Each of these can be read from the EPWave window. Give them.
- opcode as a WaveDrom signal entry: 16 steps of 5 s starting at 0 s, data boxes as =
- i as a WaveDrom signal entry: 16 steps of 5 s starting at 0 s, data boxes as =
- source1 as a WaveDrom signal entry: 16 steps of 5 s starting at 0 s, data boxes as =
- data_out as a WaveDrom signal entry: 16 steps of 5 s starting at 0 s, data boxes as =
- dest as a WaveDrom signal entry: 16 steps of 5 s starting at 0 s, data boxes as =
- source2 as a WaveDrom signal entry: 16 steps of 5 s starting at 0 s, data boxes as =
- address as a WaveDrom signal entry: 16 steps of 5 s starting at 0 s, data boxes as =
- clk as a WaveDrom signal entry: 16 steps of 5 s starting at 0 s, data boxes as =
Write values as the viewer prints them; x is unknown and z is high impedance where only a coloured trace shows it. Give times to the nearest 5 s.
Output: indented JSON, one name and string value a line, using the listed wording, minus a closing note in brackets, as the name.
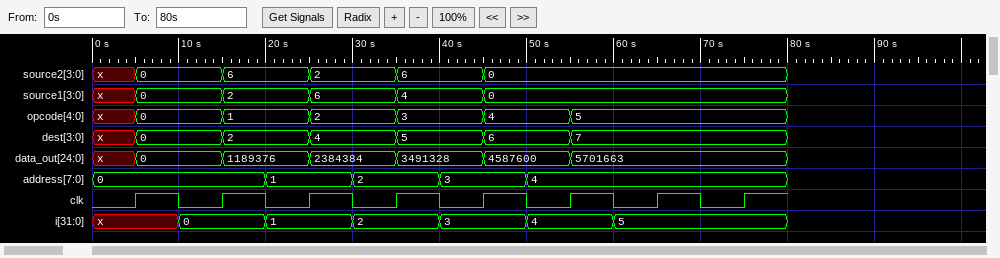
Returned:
{
  "opcode as a WaveDrom signal entry: 16 steps of 5 s starting at 0 s, data boxes as =": "{name: 'opcode', wave: 'x=.=.=.=.=.=....', data: '0 1 2 3 4 5'}",
  "i as a WaveDrom signal entry: 16 steps of 5 s starting at 0 s, data boxes as =": "{name: 'i', wave: 'x.=.=.=.=.=.=...', data: '0 1 2 3 4 5'}",
  "source1 as a WaveDrom signal entry: 16 steps of 5 s starting at 0 s, data boxes as =": "{name: 'source1', wave: 'x=.=.=.=.=......', data: '0 2 6 4 0'}",
  "data_out as a WaveDrom signal entry: 16 steps of 5 s starting at 0 s, data boxes as =": "{name: 'data_out', wave: 'x=.=.=.=.=.=....', data: '0 1189376 2384384 3491328 4587600 5701663'}",
  "dest as a WaveDrom signal entry: 16 steps of 5 s starting at 0 s, data boxes as =": "{name: 'dest', wave: 'x=.=.=.=.=.=....', data: '0 2 4 5 6 7'}",
  "source2 as a WaveDrom signal entry: 16 steps of 5 s starting at 0 s, data boxes as =": "{name: 'source2', wave: 'x=.=.=.=.=......', data: '0 6 2 6 0'}",
  "address as a WaveDrom signal entry: 16 steps of 5 s starting at 0 s, data boxes as =": "{name: 'address', wave: '=...=.=.=.=.....', data: '0 1 2 3 4'}",
  "clk as a WaveDrom signal entry: 16 steps of 5 s starting at 0 s, data boxes as =": "{name: 'clk', wave: '0101010101010101'}"
}
